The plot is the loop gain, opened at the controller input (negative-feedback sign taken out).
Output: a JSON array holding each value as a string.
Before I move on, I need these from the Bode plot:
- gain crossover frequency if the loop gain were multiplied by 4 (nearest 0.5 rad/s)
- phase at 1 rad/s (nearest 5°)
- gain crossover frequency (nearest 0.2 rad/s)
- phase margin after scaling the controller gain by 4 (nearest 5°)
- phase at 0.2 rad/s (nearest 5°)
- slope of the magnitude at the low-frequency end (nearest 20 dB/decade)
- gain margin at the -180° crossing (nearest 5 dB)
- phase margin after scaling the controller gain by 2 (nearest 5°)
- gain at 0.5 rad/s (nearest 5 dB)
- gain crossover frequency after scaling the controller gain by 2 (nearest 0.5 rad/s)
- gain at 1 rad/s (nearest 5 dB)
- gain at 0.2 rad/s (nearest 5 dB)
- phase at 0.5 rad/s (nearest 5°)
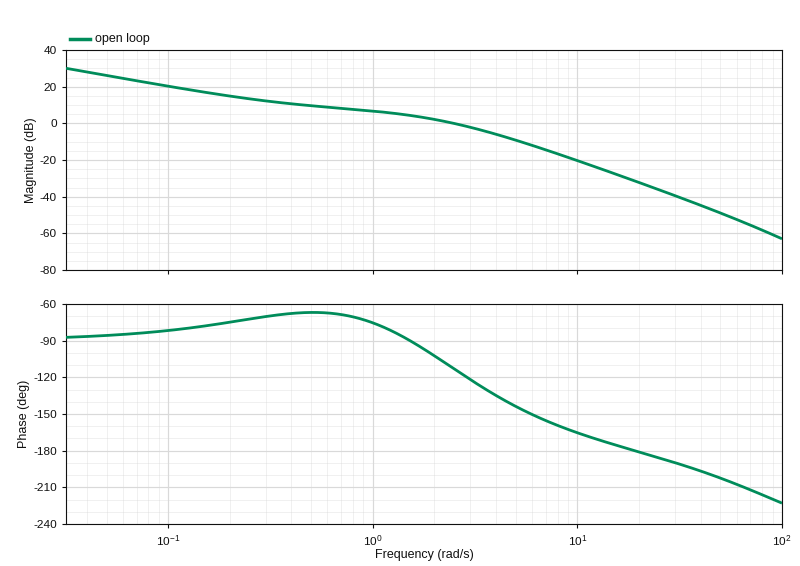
["6.0 rad/s", "-75°", "2.4 rad/s", "30°", "-75°", "-20 dB/decade", "30 dB", "45°", "10 dB", "4.0 rad/s", "5 dB", "15 dB", "-65°"]
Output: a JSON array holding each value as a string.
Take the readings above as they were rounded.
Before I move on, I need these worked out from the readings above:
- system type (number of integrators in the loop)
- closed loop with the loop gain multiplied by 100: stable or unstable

["1", "unstable"]
